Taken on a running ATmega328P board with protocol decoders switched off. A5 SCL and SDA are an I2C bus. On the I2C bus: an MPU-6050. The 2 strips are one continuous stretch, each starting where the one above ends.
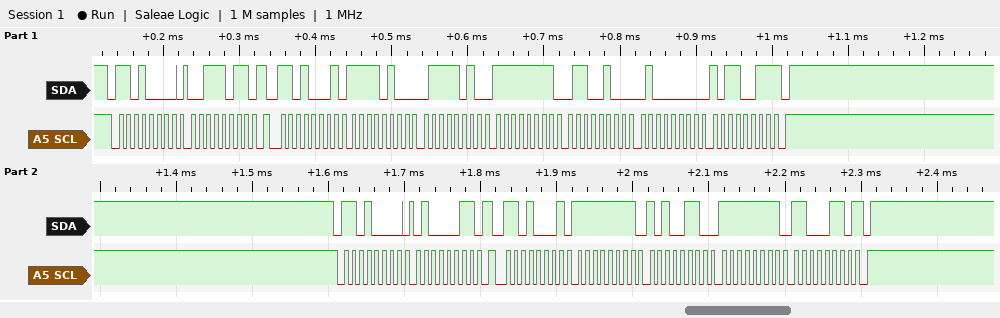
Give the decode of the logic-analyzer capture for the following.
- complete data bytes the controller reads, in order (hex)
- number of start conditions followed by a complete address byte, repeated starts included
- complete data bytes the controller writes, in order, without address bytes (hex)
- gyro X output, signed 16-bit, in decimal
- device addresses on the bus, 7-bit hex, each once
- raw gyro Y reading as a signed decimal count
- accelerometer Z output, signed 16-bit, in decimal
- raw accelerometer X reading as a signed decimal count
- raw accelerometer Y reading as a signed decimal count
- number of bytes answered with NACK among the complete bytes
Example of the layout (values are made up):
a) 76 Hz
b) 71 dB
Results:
a) F4 7A FF 64 40 B3 FF A6 FF C6
b) 4
c) 3B 43
d) -90
e) 0x68
f) -58
g) 16563
h) -2950
i) -156
j) 2
